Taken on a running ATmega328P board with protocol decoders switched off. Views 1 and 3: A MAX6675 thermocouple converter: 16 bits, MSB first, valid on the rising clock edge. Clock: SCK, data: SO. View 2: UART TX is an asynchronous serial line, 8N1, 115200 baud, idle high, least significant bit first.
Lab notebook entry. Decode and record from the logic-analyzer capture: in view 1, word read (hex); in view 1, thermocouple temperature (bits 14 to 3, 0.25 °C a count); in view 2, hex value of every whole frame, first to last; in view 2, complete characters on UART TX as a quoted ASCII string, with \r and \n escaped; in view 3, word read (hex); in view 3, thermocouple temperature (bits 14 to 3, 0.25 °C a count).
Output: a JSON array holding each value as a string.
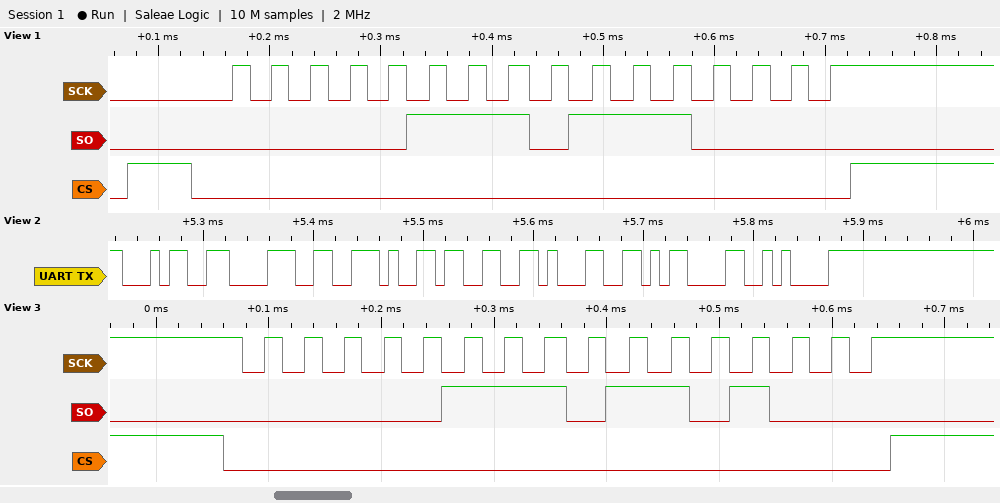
["0x0770", "59.50 °C", "34 38 2E 33 31 0D 0A", "\"48.31\\r\\n\"", "0x0768", "59.25 °C"]
